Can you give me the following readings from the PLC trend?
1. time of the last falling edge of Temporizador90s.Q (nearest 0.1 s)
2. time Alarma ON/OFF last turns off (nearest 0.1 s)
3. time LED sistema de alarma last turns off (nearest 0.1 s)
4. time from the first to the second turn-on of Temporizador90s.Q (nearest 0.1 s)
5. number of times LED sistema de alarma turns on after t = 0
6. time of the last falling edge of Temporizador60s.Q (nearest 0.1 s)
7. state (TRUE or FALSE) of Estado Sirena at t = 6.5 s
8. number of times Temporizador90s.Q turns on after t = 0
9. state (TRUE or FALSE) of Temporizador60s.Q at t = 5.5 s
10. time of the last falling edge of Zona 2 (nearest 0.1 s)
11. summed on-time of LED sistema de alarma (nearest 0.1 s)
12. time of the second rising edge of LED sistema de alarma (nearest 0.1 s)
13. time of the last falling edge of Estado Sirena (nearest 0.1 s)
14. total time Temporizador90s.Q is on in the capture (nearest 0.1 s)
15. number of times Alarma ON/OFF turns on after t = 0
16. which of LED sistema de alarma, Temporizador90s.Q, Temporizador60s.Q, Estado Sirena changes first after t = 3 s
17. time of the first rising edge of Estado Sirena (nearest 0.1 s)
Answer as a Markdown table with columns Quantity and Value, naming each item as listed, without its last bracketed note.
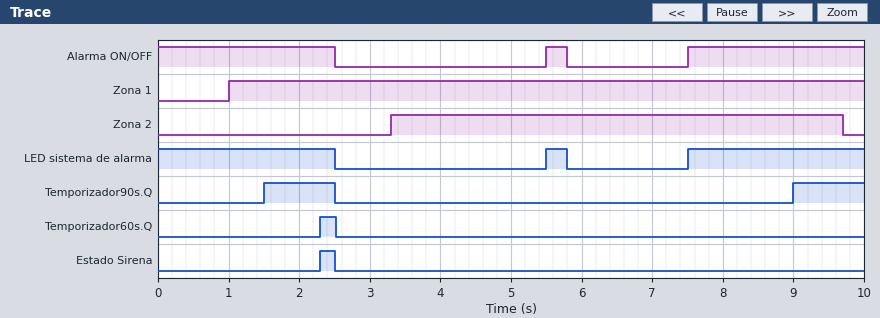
| Quantity | Value |
|---|---|
| time of the last falling edge of Temporizador90s.Q | 2.5 s |
| time Alarma ON/OFF last turns off | 5.8 s |
| time LED sistema de alarma last turns off | 5.8 s |
| time from the first to the second turn-on of Temporizador90s.Q | 7.5 s |
| number of times LED sistema de alarma turns on after t = 0 | 2 |
| time of the last falling edge of Temporizador60s.Q | 2.5 s |
| state (TRUE or FALSE) of Estado Sirena at t = 6.5 s | FALSE |
| number of times Temporizador90s.Q turns on after t = 0 | 2 |
| state (TRUE or FALSE) of Temporizador60s.Q at t = 5.5 s | FALSE |
| time of the last falling edge of Zona 2 | 9.7 s |
| summed on-time of LED sistema de alarma | 5.3 s |
| time of the second rising edge of LED sistema de alarma | 7.5 s |
| time of the last falling edge of Estado Sirena | 2.5 s |
| total time Temporizador90s.Q is on in the capture | 2.0 s |
| number of times Alarma ON/OFF turns on after t = 0 | 2 |
| which of LED sistema de alarma, Temporizador90s.Q, Temporizador60s.Q, Estado Sirena changes first after t = 3 s | LED sistema de alarma |
| time of the first rising edge of Estado Sirena | 2.3 s |
